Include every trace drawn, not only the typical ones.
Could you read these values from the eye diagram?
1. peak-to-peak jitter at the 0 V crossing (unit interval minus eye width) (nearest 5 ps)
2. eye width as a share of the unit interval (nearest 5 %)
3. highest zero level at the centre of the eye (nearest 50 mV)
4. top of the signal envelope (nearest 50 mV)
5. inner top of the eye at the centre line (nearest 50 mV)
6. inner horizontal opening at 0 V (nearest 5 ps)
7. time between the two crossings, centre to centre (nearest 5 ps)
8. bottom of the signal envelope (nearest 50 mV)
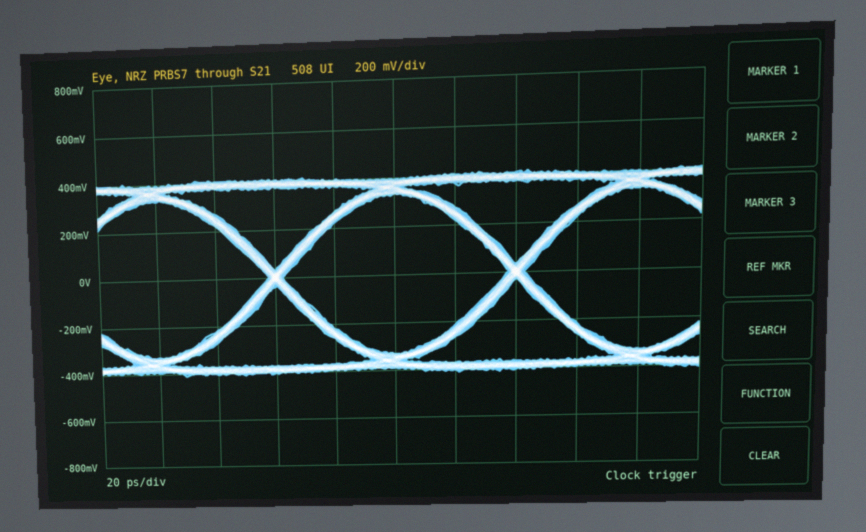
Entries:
5 ps
95 %
-350 mV
400 mV
350 mV
75 ps
80 ps
-400 mV
